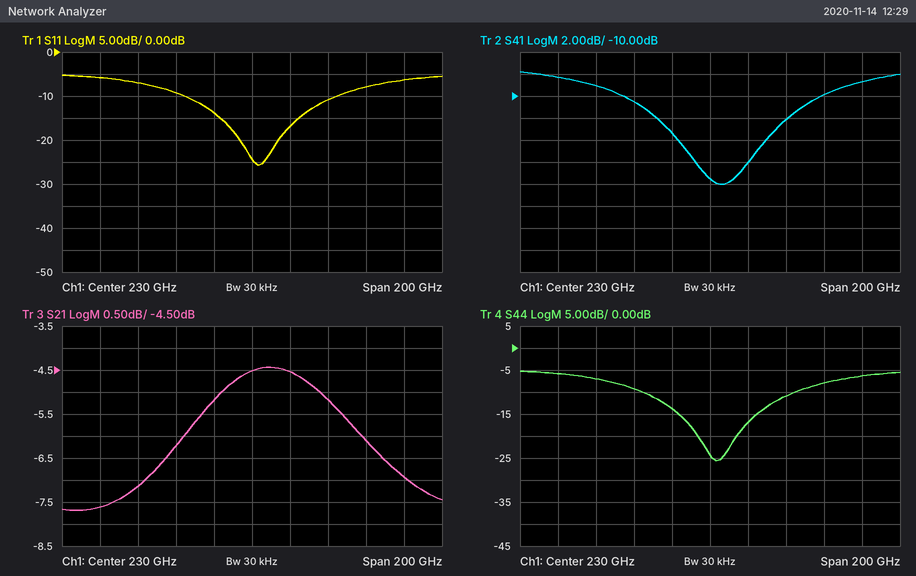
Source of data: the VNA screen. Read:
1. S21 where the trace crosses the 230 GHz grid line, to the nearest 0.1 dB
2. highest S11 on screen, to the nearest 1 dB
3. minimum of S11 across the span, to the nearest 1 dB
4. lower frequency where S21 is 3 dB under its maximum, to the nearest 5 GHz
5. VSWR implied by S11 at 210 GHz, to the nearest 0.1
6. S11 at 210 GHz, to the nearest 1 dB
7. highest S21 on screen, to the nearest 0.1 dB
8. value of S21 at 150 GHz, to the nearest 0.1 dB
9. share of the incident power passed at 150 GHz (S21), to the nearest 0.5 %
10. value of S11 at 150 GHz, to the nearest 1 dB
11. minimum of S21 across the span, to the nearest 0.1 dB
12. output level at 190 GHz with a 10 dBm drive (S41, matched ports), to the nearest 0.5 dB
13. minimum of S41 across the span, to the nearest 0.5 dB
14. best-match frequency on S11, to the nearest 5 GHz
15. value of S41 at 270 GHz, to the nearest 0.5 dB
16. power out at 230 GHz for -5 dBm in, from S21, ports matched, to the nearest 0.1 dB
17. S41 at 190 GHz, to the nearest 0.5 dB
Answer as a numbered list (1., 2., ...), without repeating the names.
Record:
1. -4.5 dB
2. -5 dB
3. -26 dB
4. 160 GHz
5. 1.5
6. -14 dB
7. -4.4 dB
8. -7.6 dB
9. 17.5 %
10. -6 dB
11. -7.7 dB
12. -0.5 dBm
13. -18.0 dB
14. 235 GHz
15. -12.0 dB
16. -9.5 dBm
17. -10.5 dB
